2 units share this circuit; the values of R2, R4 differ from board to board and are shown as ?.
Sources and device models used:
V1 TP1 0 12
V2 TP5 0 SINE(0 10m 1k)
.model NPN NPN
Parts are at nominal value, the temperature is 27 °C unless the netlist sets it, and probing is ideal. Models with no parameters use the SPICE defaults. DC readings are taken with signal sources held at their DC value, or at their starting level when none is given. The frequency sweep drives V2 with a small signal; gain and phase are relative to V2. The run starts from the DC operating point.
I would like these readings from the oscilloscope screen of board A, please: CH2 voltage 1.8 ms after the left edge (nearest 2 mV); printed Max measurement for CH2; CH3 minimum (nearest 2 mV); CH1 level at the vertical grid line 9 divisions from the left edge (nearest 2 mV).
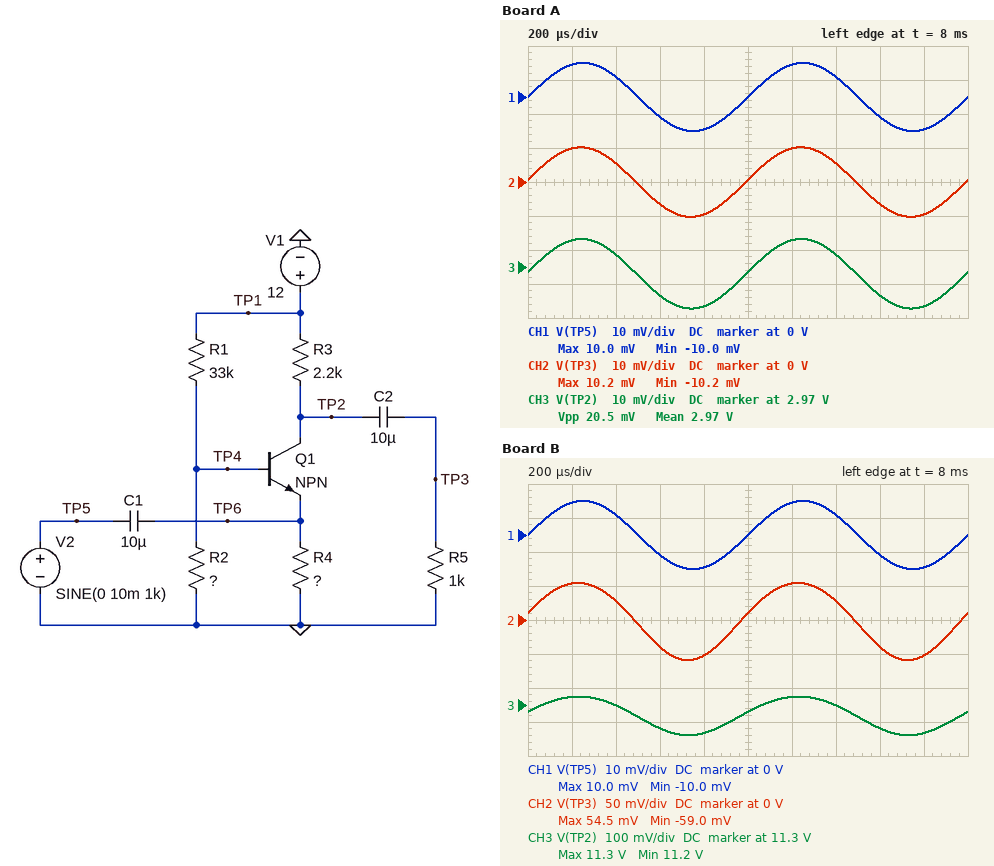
-10 mV
10.2 mV
2.958 V
-10 mV
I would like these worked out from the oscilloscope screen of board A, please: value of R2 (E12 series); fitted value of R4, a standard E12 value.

22 kΩ
680 Ω
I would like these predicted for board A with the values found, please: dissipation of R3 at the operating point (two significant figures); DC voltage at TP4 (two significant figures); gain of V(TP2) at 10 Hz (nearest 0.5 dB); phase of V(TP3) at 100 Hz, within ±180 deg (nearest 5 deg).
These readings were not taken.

37 mW
3.7 V
-12.0 dB
35 deg
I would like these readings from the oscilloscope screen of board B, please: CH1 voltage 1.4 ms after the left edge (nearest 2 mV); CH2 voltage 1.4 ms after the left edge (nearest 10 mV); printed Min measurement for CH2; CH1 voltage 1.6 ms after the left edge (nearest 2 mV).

6 mV
30 mV
-59.0 mV
-6 mV
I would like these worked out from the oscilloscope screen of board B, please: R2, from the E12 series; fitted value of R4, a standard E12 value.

4.7 kΩ
2.2 kΩ
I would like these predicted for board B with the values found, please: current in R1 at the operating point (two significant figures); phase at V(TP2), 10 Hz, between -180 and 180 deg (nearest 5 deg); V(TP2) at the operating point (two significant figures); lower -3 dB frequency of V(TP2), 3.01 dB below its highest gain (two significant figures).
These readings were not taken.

320 µA
55 deg
11 V
140 Hz
